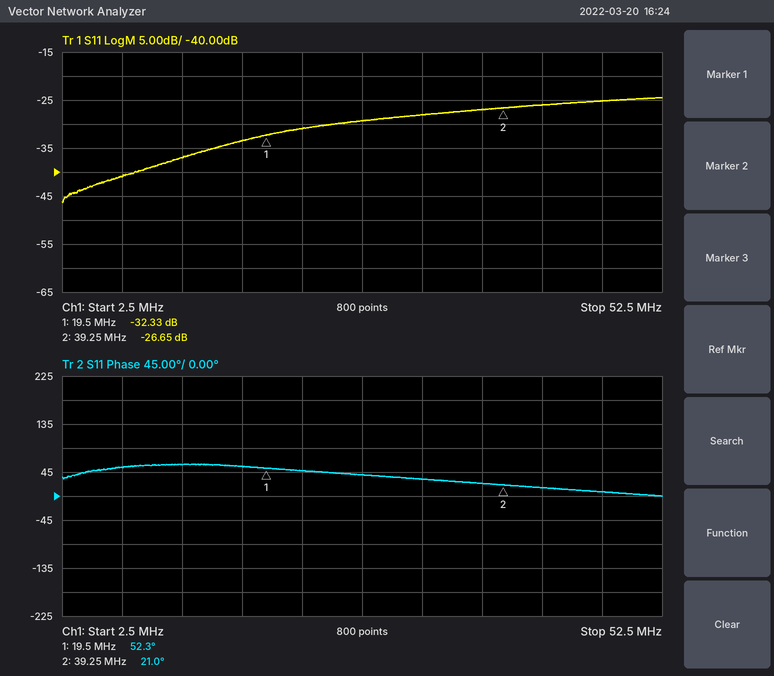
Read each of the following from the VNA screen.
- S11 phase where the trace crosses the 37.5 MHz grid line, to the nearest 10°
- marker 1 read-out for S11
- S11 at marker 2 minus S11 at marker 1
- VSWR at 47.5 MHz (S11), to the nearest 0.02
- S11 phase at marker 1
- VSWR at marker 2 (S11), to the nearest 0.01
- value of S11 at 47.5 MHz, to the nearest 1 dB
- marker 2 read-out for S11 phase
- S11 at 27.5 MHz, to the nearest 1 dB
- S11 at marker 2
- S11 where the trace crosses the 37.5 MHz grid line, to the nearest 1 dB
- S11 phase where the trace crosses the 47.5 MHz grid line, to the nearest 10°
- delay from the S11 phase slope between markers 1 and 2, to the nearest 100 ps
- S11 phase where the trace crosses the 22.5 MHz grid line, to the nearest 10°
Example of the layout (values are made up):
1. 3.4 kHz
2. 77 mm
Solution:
1. 20°
2. -32.33 dB
3. 5.68 dB
4. 1.12
5. 52.3°
6. 1.10
7. -25 dB
8. 21.0°
9. -29 dB
10. -26.65 dB
11. -27 dB
12. 10°
13. 4.4 ns
14. 50°
